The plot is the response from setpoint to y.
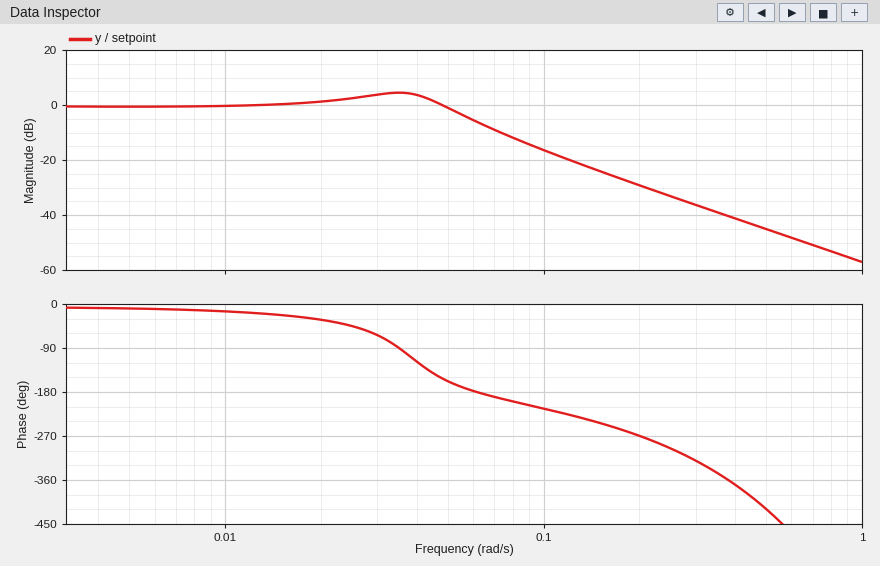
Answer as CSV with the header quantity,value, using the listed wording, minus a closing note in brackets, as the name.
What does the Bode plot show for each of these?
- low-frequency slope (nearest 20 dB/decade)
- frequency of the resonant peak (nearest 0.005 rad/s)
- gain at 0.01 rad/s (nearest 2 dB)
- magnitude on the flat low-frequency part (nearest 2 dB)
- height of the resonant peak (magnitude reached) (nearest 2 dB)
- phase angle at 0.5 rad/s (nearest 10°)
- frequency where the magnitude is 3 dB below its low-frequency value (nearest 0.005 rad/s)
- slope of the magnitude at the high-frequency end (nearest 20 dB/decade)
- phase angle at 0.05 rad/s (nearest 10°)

quantity,value
low-frequency slope,0 dB/decade
frequency of the resonant peak,0.035 rad/s
gain at 0.01 rad/s,0 dB
magnitude on the flat low-frequency part,0 dB
height of the resonant peak (magnitude reached),4 dB
phase angle at 0.5 rad/s,-420°
frequency where the magnitude is 3 dB below its low-frequency value,0.055 rad/s
slope of the magnitude at the high-frequency end,-40 dB/decade
phase angle at 0.05 rad/s,-160°
